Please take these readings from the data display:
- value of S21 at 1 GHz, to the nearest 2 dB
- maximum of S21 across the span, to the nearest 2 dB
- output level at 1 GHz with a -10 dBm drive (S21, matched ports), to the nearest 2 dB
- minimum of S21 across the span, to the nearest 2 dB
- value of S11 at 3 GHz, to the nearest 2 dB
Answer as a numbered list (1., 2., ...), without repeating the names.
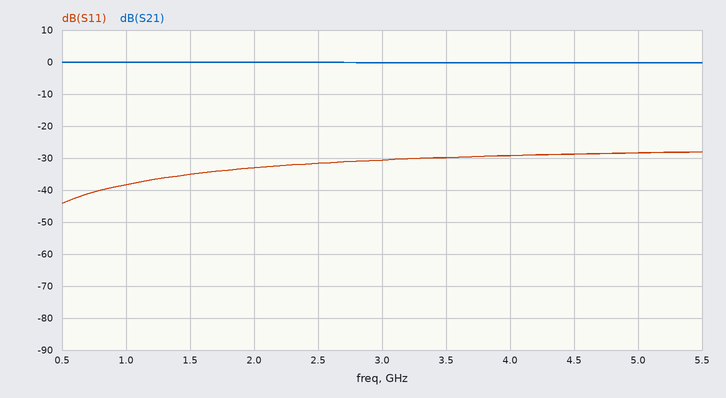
1. 0 dB
2. 0 dB
3. -10 dBm
4. 0 dB
5. -30 dB
